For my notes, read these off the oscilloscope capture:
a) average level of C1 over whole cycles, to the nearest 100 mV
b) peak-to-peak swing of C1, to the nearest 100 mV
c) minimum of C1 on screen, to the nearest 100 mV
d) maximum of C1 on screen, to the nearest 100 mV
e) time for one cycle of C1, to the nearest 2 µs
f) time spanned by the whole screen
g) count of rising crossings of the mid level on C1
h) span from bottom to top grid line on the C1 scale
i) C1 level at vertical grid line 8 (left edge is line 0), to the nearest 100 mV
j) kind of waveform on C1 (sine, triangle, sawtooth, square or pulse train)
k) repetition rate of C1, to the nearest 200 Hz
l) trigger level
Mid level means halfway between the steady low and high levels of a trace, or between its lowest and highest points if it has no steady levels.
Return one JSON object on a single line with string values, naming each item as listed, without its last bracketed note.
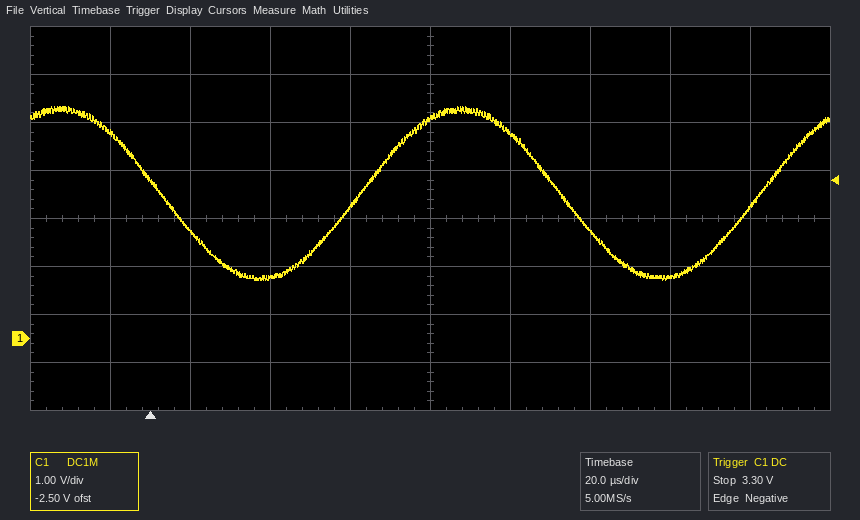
{"average level of C1 over whole cycles, to the nearest 100 mV": "3.0 V", "peak-to-peak swing of C1, to the nearest 100 mV": "3.6 V", "minimum of C1 on screen, to the nearest 100 mV": "1.2 V", "maximum of C1 on screen, to the nearest 100 mV": "4.8 V", "time for one cycle of C1, to the nearest 2 µs": "100 µs", "time spanned by the whole screen": "200 µs", "count of rising crossings of the mid level on C1": "2", "span from bottom to top grid line on the C1 scale": "8 V", "C1 level at vertical grid line 8 (left edge is line 0), to the nearest 100 mV": "1.3 V", "kind of waveform on C1": "sine", "repetition rate of C1, to the nearest 200 Hz": "10.0 kHz", "trigger level": "3.30 V"}
